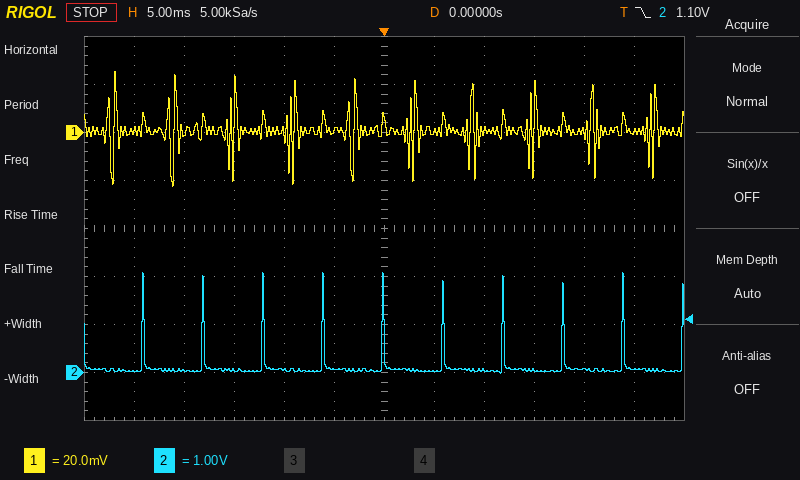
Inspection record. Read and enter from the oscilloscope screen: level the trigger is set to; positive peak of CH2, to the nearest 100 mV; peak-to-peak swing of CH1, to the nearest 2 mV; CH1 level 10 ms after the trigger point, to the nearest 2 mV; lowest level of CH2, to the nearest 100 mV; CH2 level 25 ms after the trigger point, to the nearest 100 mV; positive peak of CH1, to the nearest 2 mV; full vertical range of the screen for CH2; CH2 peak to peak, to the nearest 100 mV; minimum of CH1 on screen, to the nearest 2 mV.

1.10 V
2.1 V
48 mV
0 mV
0.0 V
100 mV
26 mV
8 V
2.1 V
-22 mV
